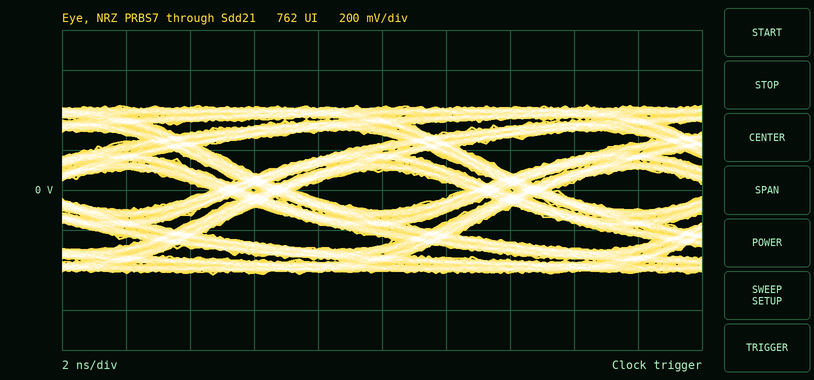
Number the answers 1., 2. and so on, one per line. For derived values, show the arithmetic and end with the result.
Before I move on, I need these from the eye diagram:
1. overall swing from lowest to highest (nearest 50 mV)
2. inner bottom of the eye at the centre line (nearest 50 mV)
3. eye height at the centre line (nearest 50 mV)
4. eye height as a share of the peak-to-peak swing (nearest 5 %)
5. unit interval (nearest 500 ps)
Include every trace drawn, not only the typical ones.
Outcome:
1. 850 mV
2. -100 mV
3. 200 mV
4. 200 mV / 850 mV ≈ 23.5 %, so 25 % to the nearest 5 %
5. 8.0 ns
